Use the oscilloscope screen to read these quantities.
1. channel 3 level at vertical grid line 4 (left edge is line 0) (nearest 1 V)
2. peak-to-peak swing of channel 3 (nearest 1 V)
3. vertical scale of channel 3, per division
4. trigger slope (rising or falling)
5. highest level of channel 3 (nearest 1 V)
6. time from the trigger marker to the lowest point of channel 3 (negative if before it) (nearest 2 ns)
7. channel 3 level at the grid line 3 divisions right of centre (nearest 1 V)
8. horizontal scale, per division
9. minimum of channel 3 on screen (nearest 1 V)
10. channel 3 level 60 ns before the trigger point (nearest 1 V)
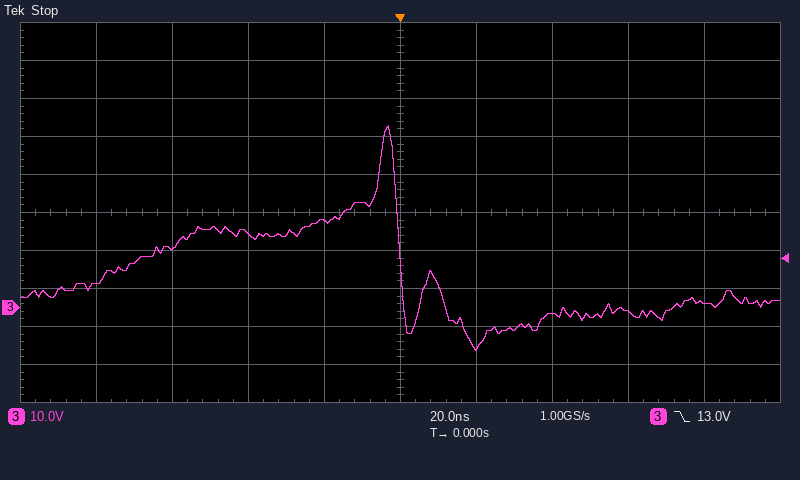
23 V
59 V
10 V
falling
48 V
+20 ns
-1 V
20 ns
-11 V
16 V
